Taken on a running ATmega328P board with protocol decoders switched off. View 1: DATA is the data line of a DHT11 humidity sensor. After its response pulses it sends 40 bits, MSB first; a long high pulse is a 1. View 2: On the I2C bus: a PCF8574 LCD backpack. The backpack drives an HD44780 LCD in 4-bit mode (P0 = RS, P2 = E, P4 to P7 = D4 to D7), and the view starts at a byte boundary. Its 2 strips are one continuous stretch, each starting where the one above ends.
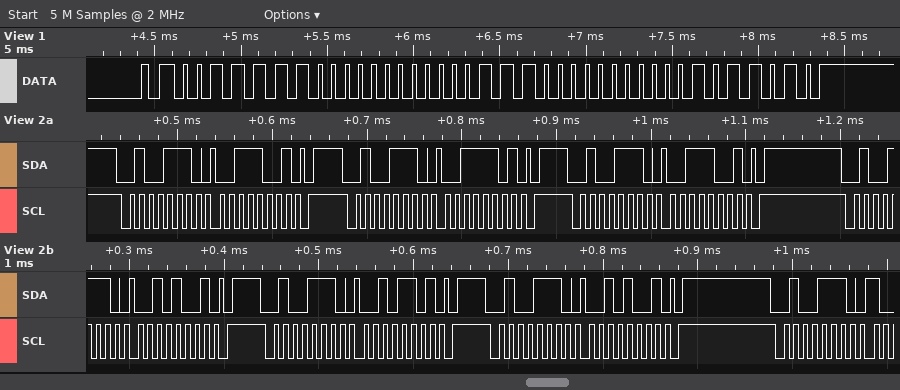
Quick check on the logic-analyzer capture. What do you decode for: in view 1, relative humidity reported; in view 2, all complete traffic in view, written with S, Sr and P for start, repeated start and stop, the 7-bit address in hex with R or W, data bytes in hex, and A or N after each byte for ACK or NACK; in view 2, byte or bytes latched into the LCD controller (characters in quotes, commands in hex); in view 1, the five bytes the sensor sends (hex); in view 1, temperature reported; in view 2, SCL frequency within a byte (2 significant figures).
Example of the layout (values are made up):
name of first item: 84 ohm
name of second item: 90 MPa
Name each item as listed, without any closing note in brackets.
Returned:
in view 1, relative humidity reported: 62 %
in view 2, all complete traffic in view, written with S, Sr and P for start, repeated start and stop, the 7-bit address in hex with R or W, data bytes in hex, and A or N after each byte for ACK or NACK: S 27W A 39 A P S 27W A 3D A P S 27W A 39 A P S 27W A 29 A P S 27W A 2D A P S 27W A 29 A P S 27W A
in view 2, byte or bytes latched into the LCD controller: '2'
in view 1, the five bytes the sensor sends: 3E 00 1C 00 5A
in view 1, temperature reported: 28.0 °C
in view 2, SCL frequency within a byte: 100 kHz
